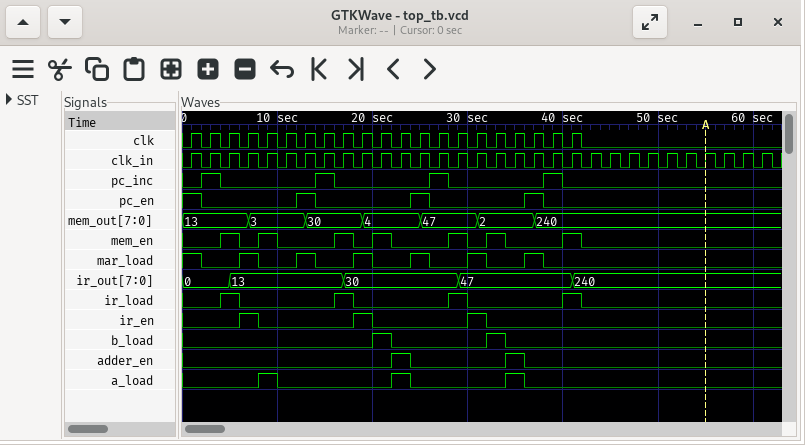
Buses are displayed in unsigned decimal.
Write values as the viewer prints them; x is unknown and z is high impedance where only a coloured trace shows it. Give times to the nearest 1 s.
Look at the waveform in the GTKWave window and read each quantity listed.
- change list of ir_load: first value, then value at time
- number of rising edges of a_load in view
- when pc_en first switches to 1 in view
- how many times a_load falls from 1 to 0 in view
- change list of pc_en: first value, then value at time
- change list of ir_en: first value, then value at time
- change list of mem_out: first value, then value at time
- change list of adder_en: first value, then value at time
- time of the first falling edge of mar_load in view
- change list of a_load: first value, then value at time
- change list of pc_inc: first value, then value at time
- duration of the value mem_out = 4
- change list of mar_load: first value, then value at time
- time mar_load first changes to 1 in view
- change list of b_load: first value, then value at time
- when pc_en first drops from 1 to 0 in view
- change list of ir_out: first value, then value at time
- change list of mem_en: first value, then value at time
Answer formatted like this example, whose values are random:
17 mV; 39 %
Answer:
0, 1 at 4 s, 0 at 6 s, 1 at 16 s, 0 at 18 s, 1 at 28 s, 0 at 30 s, 1 at 40 s, 0 at 42 s; 3; 12 s; 3; 1, 0 at 2 s, 1 at 12 s, 0 at 14 s, 1 at 24 s, 0 at 26 s, 1 at 36 s, 0 at 38 s; 0, 1 at 6 s, 0 at 8 s, 1 at 18 s, 0 at 20 s, 1 at 30 s, 0 at 32 s; 13, 3 at 7 s, 30 at 13 s, 4 at 19 s, 47 at 25 s, 2 at 31 s, 240 at 37 s; 0, 1 at 22 s, 0 at 24 s, 1 at 34 s, 0 at 36 s; 2 s; 0, 1 at 8 s, 0 at 10 s, 1 at 22 s, 0 at 24 s, 1 at 34 s, 0 at 36 s; 0, 1 at 2 s, 0 at 4 s, 1 at 14 s, 0 at 16 s, 1 at 26 s, 0 at 28 s, 1 at 38 s, 0 at 40 s; 6 s; 1, 0 at 2 s, 1 at 6 s, 0 at 8 s, 1 at 12 s, 0 at 14 s, 1 at 18 s, 0 at 20 s, 1 at 24 s, 0 at 26 s, 1 at 30 s, 0 at 32 s, 1 at 36 s, 0 at 38 s; 6 s; 0, 1 at 20 s, 0 at 22 s, 1 at 32 s, 0 at 34 s; 2 s; 0, 13 at 5 s, 30 at 17 s, 47 at 29 s, 240 at 41 s; 0, 1 at 4 s, 0 at 6 s, 1 at 8 s, 0 at 10 s, 1 at 16 s, 0 at 18 s, 1 at 20 s, 0 at 22 s, 1 at 28 s, 0 at 30 s, 1 at 32 s, 0 at 34 s, 1 at 40 s, 0 at 42 s
